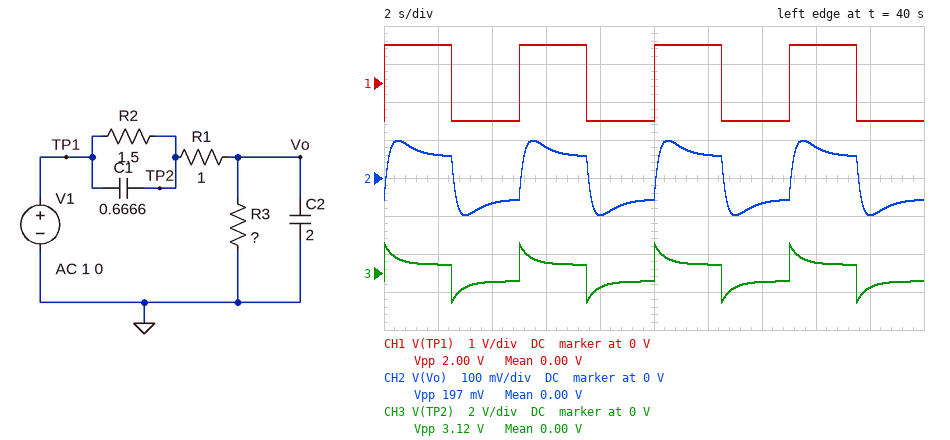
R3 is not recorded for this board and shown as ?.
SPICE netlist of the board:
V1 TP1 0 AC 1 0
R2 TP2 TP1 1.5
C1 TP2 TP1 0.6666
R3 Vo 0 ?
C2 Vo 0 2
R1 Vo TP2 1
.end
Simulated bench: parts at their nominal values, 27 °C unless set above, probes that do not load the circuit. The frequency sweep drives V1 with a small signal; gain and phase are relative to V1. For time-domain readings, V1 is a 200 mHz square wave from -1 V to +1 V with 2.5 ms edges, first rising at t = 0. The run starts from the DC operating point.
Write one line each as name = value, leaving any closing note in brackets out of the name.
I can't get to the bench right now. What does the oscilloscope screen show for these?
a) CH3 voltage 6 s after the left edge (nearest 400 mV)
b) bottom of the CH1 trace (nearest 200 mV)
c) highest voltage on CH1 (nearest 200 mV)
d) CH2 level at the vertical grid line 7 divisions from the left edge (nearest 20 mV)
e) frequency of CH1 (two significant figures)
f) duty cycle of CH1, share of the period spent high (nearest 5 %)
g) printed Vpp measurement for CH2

CH3 voltage 6 s after the left edge = 400 mV
bottom of the CH1 trace = -1.0 V
highest voltage on CH1 = 1.0 V
CH2 level at the vertical grid line 7 divisions from the left edge = -60 mV
frequency of CH1 = 200 mHz
duty cycle of CH1, share of the period spent high = 50 %
printed Vpp measurement for CH2 = 197 mV
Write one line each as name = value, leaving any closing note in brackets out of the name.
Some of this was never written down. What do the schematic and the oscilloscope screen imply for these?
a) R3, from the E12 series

R3, from the E12 series = 0.15 Ω
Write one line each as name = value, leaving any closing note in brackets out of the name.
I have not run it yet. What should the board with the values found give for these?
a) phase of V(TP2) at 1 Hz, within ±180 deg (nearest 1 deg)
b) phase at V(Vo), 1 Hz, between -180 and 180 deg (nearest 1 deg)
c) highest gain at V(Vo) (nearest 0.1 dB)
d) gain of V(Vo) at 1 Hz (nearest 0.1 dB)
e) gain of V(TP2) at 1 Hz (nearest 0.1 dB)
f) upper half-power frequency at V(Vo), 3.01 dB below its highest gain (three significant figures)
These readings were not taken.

phase of V(TP2) at 1 Hz, within ±180 deg = 12 deg
phase at V(Vo), 1 Hz, between -180 and 180 deg = -47 deg
highest gain at V(Vo) = -21.5 dB
gain of V(Vo) at 1 Hz = -24.0 dB
gain of V(TP2) at 1 Hz = -0.6 dB
upper half-power frequency at V(Vo), 3.01 dB below its highest gain = 1.11 Hz
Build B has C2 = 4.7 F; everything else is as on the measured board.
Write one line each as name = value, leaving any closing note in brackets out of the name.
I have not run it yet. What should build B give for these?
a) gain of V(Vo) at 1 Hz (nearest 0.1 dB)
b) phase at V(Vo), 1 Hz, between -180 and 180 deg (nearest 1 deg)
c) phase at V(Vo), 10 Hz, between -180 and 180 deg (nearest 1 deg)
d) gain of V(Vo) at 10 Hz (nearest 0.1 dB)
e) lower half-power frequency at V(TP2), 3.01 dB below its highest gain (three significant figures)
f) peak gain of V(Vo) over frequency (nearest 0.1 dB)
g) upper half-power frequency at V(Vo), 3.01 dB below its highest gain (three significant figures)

gain of V(Vo) at 1 Hz = -30.3 dB
phase at V(Vo), 1 Hz, between -180 and 180 deg = -63 deg
phase at V(Vo), 10 Hz, between -180 and 180 deg = -87 deg
gain of V(Vo) at 10 Hz = -49.4 dB
lower half-power frequency at V(TP2), 3.01 dB below its highest gain = 329 mHz
peak gain of V(Vo) over frequency = -24.3 dB
upper half-power frequency at V(Vo), 3.01 dB below its highest gain = 630 mHz
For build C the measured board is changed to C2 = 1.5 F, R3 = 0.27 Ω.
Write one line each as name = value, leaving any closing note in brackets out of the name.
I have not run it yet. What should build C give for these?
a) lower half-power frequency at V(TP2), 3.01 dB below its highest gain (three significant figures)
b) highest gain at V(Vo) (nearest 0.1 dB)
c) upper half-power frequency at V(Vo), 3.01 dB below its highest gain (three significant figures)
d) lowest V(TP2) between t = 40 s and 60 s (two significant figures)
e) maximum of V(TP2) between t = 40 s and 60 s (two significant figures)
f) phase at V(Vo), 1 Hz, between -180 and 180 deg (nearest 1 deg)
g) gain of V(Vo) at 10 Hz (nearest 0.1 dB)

lower half-power frequency at V(TP2), 3.01 dB below its highest gain = 307 mHz
highest gain at V(Vo) = -17.8 dB
upper half-power frequency at V(Vo), 3.01 dB below its highest gain = 956 mHz
lowest V(TP2) between t = 40 s and 60 s = -1.5 V
maximum of V(TP2) between t = 40 s and 60 s = 1.5 V
phase at V(Vo), 1 Hz, between -180 and 180 deg = -52 deg
gain of V(Vo) at 10 Hz = -39.5 dB
